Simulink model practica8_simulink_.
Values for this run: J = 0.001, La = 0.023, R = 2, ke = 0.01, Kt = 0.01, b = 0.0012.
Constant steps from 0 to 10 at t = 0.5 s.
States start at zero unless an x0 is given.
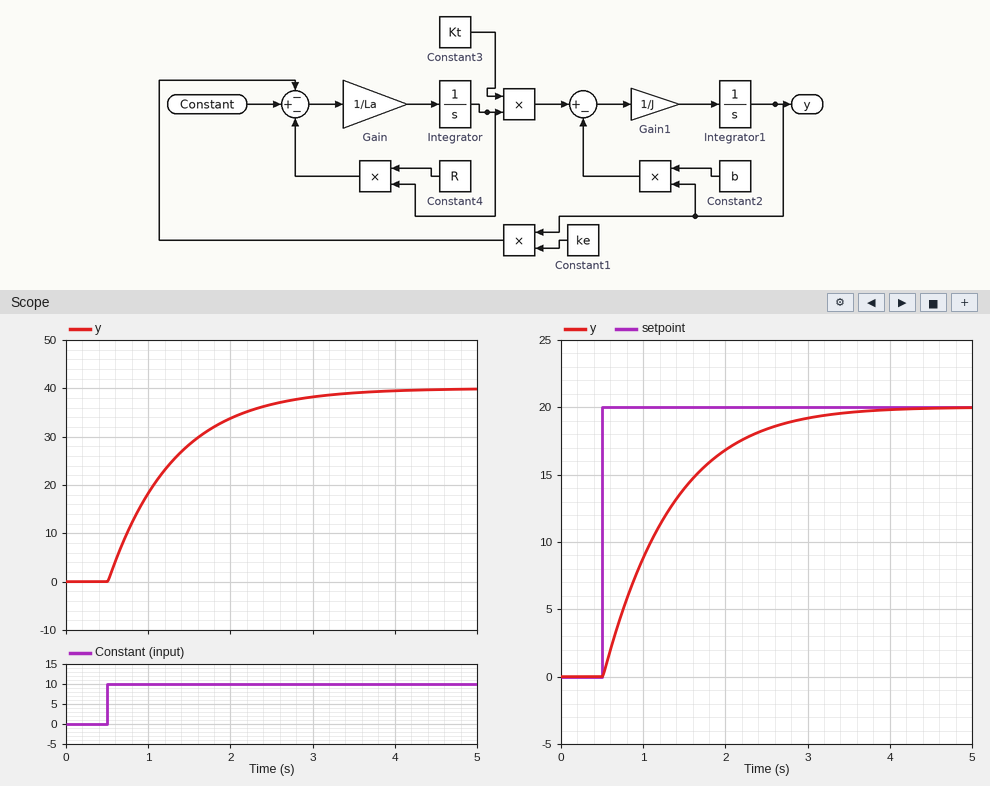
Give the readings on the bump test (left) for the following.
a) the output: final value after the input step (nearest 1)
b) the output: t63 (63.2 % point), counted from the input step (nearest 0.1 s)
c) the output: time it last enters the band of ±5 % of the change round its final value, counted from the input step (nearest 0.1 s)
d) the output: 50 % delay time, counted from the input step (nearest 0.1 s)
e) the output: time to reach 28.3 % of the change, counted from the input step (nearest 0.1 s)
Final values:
40
0.8 s
2.4 s
0.6 s
0.3 s
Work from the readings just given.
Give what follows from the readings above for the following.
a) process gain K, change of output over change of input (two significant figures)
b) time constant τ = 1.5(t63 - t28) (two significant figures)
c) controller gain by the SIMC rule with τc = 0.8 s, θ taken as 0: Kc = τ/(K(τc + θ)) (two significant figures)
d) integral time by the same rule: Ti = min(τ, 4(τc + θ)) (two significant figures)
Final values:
4.0
0.75 s
0.23
0.75 s
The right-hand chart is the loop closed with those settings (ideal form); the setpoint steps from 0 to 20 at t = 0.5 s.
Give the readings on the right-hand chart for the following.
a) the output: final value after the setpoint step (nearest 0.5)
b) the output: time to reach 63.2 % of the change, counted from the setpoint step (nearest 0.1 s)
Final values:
20.0
0.8 s
